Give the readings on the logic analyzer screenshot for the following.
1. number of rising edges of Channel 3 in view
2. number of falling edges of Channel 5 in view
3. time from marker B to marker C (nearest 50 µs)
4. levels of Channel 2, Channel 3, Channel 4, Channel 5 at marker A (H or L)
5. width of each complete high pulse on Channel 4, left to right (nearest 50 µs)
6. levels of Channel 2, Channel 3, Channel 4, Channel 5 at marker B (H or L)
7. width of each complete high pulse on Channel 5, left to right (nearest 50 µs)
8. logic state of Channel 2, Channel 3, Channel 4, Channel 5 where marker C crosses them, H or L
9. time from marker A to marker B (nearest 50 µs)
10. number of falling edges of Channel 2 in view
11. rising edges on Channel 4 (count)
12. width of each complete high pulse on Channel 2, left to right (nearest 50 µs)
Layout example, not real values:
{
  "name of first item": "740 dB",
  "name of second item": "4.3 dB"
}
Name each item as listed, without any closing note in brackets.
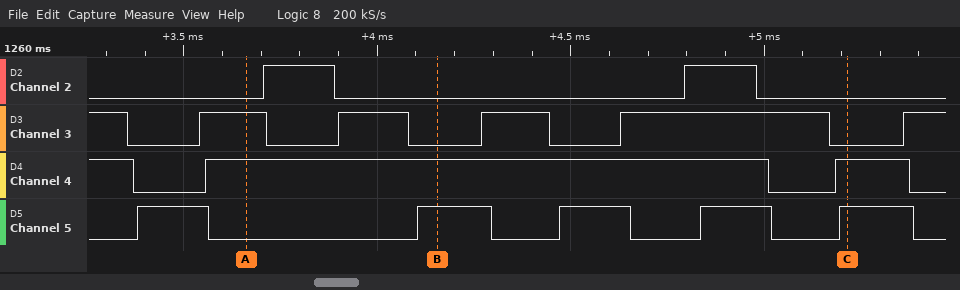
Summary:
{
  "number of rising edges of Channel 3 in view": "5",
  "number of falling edges of Channel 5 in view": "5",
  "time from marker B to marker C": "1050 µs",
  "levels of Channel 2, Channel 3, Channel 4, Channel 5 at marker A": "Channel 2=L, Channel 3=H, Channel 4=H, Channel 5=L",
  "width of each complete high pulse on Channel 4, left to right": "1450 µs, 200 µs",
  "levels of Channel 2, Channel 3, Channel 4, Channel 5 at marker B": "Channel 2=L, Channel 3=L, Channel 4=H, Channel 5=H",
  "width of each complete high pulse on Channel 5, left to right": "200 µs, 200 µs, 200 µs, 200 µs, 200 µs",
  "logic state of Channel 2, Channel 3, Channel 4, Channel 5 where marker C crosses them, H or L": "Channel 2=L, Channel 3=L, Channel 4=H, Channel 5=H",
  "time from marker A to marker B": "500 µs",
  "number of falling edges of Channel 2 in view": "2",
  "rising edges on Channel 4": "2",
  "width of each complete high pulse on Channel 2, left to right": "200 µs, 200 µs"
}
